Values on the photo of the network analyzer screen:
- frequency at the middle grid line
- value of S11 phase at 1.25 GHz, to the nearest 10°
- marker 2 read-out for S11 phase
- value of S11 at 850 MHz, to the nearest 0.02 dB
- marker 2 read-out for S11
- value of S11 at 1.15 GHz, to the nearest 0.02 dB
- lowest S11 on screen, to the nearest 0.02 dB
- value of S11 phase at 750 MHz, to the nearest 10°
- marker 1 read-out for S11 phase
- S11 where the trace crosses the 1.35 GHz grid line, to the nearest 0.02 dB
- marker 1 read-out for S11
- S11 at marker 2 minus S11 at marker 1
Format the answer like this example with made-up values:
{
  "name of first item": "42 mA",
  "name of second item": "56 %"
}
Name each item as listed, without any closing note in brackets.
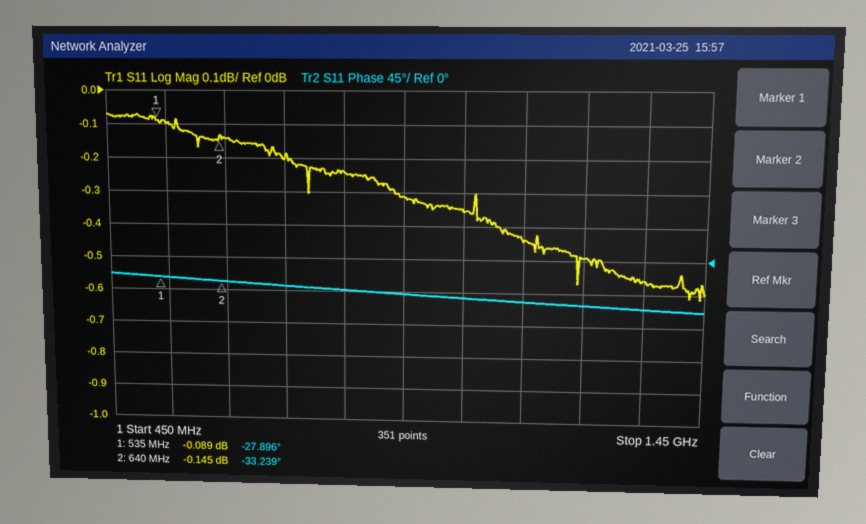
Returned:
{
  "frequency at the middle grid line": "950 MHz",
  "value of S11 phase at 1.25 GHz, to the nearest 10°": "-60°",
  "marker 2 read-out for S11 phase": "-33.239°",
  "value of S11 at 850 MHz, to the nearest 0.02 dB": "-0.24 dB",
  "marker 2 read-out for S11": "-0.145 dB",
  "value of S11 at 1.15 GHz, to the nearest 0.02 dB": "-0.44 dB",
  "lowest S11 on screen, to the nearest 0.02 dB": "-0.62 dB",
  "value of S11 phase at 750 MHz, to the nearest 10°": "-40°",
  "marker 1 read-out for S11 phase": "-27.896°",
  "S11 where the trace crosses the 1.35 GHz grid line, to the nearest 0.02 dB": "-0.56 dB",
  "marker 1 read-out for S11": "-0.089 dB",
  "S11 at marker 2 minus S11 at marker 1": "-0.056 dB"
}
